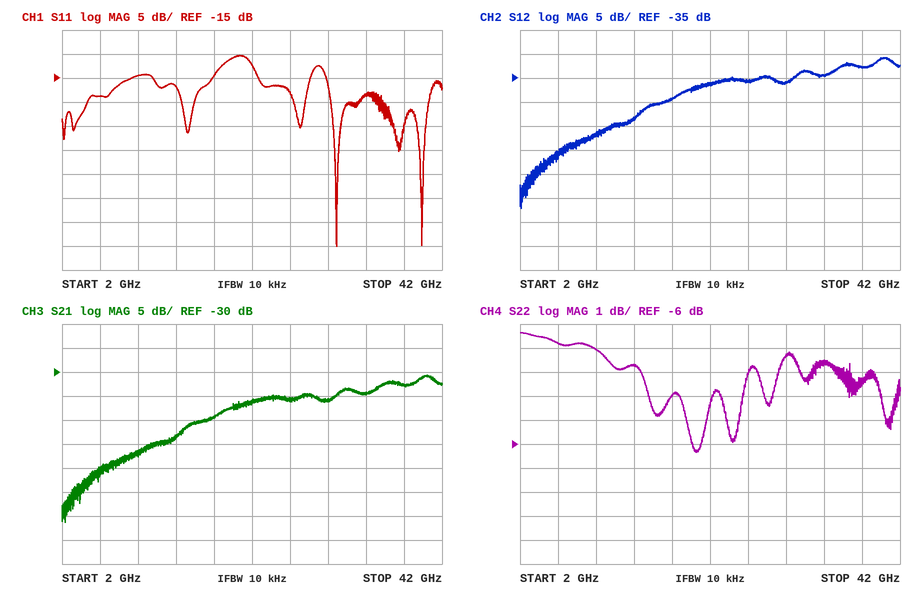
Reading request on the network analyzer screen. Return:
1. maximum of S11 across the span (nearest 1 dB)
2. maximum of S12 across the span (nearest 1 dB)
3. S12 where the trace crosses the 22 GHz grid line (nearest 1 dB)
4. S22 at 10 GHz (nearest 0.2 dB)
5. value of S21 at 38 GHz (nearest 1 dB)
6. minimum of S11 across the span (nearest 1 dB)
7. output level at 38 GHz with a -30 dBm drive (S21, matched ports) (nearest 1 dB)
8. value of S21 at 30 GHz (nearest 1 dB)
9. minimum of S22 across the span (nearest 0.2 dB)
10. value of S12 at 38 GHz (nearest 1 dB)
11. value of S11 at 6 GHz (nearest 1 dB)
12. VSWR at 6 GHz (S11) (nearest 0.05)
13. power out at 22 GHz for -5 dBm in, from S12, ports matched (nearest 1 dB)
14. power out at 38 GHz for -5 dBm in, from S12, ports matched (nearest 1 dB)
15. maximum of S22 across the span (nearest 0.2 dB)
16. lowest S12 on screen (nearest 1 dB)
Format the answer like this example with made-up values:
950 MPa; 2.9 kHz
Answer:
-10 dB; -31 dB; -36 dB; -2.0 dB; -33 dB; -50 dB; -63 dBm; -36 dB; -6.4 dB; -33 dB; -19 dB; 1.25; -41 dBm; -38 dBm; -1.4 dB; -62 dB
